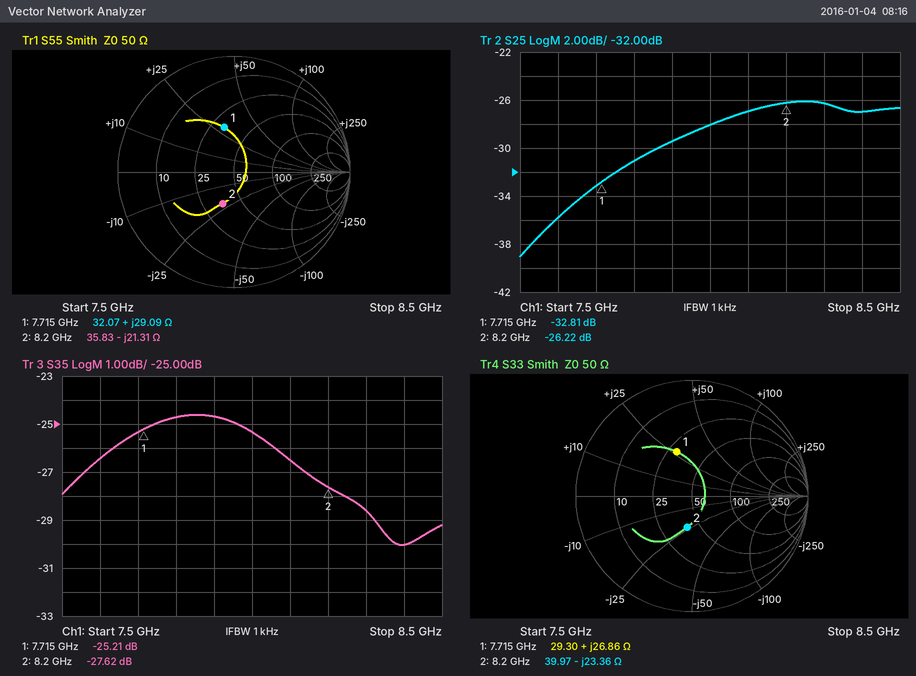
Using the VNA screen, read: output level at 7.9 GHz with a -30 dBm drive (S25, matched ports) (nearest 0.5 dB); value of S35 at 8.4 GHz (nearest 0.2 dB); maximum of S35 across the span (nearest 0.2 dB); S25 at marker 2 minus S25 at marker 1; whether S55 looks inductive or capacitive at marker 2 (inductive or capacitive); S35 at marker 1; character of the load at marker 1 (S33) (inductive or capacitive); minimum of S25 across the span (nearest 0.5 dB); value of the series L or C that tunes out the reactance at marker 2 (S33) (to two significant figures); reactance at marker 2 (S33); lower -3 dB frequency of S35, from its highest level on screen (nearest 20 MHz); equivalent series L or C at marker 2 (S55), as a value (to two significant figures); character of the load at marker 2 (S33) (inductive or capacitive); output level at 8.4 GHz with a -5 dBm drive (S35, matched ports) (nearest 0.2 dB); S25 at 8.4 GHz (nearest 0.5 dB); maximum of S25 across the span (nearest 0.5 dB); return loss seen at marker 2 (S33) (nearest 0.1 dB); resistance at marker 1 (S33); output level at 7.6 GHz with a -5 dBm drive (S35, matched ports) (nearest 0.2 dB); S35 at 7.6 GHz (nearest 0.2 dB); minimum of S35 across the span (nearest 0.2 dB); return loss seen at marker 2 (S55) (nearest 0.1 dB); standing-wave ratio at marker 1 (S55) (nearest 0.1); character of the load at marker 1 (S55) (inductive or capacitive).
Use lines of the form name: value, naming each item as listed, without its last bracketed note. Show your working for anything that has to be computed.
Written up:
output level at 7.9 GHz with a -30 dBm drive (S25, matched ports): -30 dBm + (-29.5 dB) = -59.5 dBm
value of S35 at 8.4 GHz: -30.0 dB
maximum of S35 across the span: -24.6 dB
S25 at marker 2 minus S25 at marker 1: -26.22 − (-32.81) = 6.59 dB
whether S55 looks inductive or capacitive at marker 2: capacitive
S35 at marker 1: -25.21 dB
character of the load at marker 1 (S33): inductive
minimum of S25 across the span: -39.0 dB
value of the series L or C that tunes out the reactance at marker 2 (S33): L = 23.36 Ω/(2π × 8.2 GHz) ≈ 453 pH, so 450 pH to two significant figures
reactance at marker 2: -23.36 Ω
lower -3 dB frequency of S35, from its highest level on screen: 7.52 GHz
equivalent series L or C at marker 2 (S55), as a value: C = 1/(2π × 8.2 GHz × 21.31 Ω) ≈ 911 fF, so 910 fF to two significant figures
character of the load at marker 2 (S33): capacitive
output level at 8.4 GHz with a -5 dBm drive (S35, matched ports): -5 dBm + (-30.0 dB) = -35.0 dBm
S25 at 8.4 GHz: -27.0 dB
maximum of S25 across the span: -26.0 dB
return loss seen at marker 2 (S33): 11.3 dB
resistance at marker 1: 29.30 Ω
output level at 7.6 GHz with a -5 dBm drive (S35, matched ports): -5 dBm + (-26.4 dB) = -31.4 dBm
S35 at 7.6 GHz: -26.4 dB
minimum of S35 across the span: -30.0 dB
return loss seen at marker 2 (S55): 10.8 dB
standing-wave ratio at marker 1 (S55): 2.3
character of the load at marker 1 (S55): inductive
